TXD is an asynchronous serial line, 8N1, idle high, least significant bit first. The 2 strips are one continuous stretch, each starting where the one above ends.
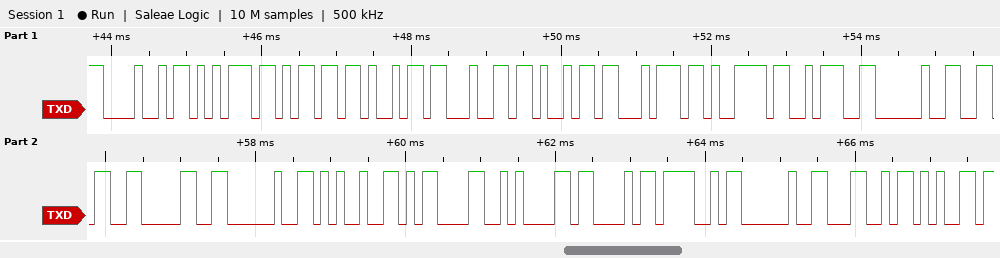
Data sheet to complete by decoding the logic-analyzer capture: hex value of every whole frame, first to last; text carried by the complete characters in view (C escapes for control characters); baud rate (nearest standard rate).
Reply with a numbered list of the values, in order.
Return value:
1. 48 75 6D 69 64 69 74 79 3A 20 36 30 20 25 0D 0A 43 4F 20 4C 65
2. "Humidity: 60 %\r\nCO Le"
3. 9600 baud
